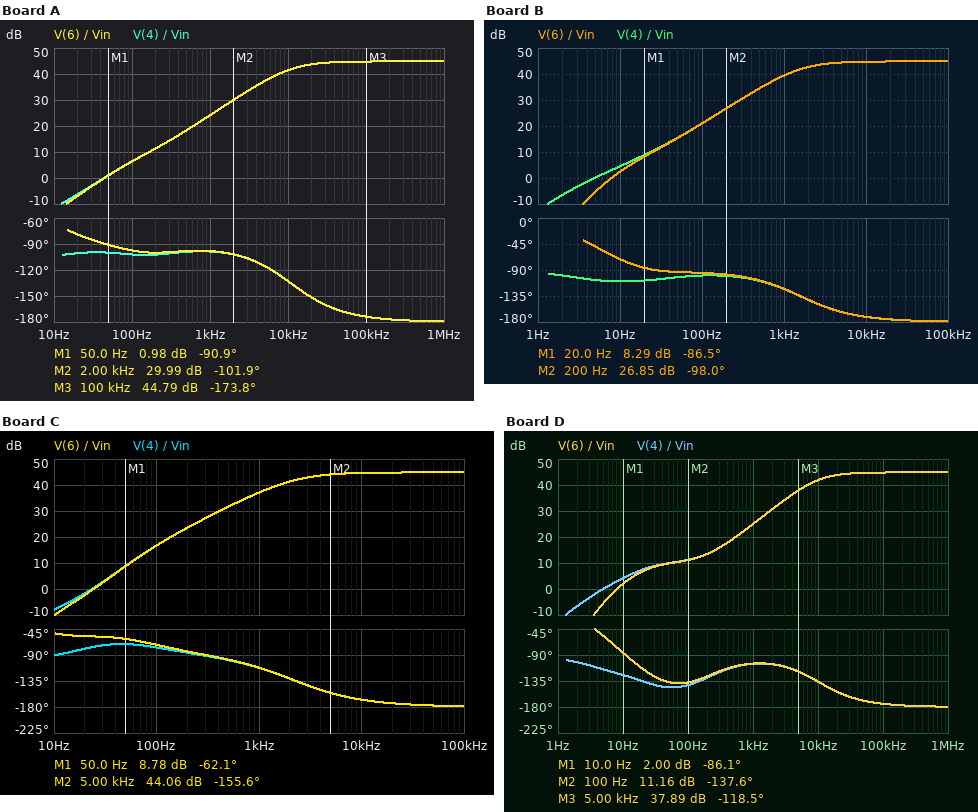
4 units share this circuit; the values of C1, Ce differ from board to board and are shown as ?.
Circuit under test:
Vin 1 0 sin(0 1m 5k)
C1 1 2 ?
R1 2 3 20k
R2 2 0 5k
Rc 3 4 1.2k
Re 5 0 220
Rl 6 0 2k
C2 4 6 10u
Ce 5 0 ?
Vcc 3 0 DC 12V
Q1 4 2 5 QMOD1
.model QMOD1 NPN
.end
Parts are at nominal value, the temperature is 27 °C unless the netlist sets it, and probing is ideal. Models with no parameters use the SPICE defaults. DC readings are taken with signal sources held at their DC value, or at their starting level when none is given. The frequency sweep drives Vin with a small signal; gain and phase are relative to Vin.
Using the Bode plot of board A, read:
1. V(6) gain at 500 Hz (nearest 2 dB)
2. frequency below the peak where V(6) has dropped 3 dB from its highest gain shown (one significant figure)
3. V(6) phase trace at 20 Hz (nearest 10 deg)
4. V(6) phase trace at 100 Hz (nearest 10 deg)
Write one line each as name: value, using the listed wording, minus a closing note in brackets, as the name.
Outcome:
V(6) gain at 500 Hz: 18 dB
frequency below the peak where V(6) has dropped 3 dB from its highest gain shown: 10 kHz
V(6) phase trace at 20 Hz: -80 deg
V(6) phase trace at 100 Hz: -100 deg
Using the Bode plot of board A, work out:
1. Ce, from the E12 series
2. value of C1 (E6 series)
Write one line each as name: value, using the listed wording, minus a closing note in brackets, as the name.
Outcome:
Ce, from the E12 series: 3.9 µF
value of C1: 330 nF
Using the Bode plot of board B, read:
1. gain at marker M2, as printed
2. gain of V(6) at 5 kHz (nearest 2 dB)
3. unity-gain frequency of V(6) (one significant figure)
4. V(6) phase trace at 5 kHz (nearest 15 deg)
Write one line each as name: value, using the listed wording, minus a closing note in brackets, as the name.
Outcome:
gain at marker M2, as printed: 26.85 dB
gain of V(6) at 5 kHz: 44 dB
unity-gain frequency of V(6): 8 Hz
V(6) phase trace at 5 kHz: -165 deg
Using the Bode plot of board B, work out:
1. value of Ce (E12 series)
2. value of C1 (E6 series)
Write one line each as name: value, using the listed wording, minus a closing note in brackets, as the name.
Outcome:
value of Ce: 27 µF
value of C1: 2.2 µF
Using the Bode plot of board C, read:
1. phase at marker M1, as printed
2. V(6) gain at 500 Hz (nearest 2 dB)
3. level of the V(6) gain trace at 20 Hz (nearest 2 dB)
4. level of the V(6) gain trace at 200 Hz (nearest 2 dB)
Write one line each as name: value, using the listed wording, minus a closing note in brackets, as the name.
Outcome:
phase at marker M1, as printed: -62.1 deg
V(6) gain at 500 Hz: 32 dB
level of the V(6) gain trace at 20 Hz: -2 dB
level of the V(6) gain trace at 200 Hz: 24 dB
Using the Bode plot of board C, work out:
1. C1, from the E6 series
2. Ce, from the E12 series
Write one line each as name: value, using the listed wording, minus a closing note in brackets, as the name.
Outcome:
C1, from the E6 series: 470 nF
Ce, from the E12 series: 27 µF
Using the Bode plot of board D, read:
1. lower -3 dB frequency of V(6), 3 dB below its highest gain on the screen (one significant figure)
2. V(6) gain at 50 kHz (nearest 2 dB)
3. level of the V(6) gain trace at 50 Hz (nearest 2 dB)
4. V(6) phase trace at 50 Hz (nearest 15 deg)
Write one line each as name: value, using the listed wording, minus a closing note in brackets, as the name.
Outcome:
lower -3 dB frequency of V(6), 3 dB below its highest gain on the screen: 10 kHz
V(6) gain at 50 kHz: 44 dB
level of the V(6) gain trace at 50 Hz: 10 dB
V(6) phase trace at 50 Hz: -135 deg
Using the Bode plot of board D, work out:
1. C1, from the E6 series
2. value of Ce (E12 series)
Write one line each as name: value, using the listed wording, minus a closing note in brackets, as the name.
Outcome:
C1, from the E6 series: 2.2 µF
value of Ce: 3.9 µF
